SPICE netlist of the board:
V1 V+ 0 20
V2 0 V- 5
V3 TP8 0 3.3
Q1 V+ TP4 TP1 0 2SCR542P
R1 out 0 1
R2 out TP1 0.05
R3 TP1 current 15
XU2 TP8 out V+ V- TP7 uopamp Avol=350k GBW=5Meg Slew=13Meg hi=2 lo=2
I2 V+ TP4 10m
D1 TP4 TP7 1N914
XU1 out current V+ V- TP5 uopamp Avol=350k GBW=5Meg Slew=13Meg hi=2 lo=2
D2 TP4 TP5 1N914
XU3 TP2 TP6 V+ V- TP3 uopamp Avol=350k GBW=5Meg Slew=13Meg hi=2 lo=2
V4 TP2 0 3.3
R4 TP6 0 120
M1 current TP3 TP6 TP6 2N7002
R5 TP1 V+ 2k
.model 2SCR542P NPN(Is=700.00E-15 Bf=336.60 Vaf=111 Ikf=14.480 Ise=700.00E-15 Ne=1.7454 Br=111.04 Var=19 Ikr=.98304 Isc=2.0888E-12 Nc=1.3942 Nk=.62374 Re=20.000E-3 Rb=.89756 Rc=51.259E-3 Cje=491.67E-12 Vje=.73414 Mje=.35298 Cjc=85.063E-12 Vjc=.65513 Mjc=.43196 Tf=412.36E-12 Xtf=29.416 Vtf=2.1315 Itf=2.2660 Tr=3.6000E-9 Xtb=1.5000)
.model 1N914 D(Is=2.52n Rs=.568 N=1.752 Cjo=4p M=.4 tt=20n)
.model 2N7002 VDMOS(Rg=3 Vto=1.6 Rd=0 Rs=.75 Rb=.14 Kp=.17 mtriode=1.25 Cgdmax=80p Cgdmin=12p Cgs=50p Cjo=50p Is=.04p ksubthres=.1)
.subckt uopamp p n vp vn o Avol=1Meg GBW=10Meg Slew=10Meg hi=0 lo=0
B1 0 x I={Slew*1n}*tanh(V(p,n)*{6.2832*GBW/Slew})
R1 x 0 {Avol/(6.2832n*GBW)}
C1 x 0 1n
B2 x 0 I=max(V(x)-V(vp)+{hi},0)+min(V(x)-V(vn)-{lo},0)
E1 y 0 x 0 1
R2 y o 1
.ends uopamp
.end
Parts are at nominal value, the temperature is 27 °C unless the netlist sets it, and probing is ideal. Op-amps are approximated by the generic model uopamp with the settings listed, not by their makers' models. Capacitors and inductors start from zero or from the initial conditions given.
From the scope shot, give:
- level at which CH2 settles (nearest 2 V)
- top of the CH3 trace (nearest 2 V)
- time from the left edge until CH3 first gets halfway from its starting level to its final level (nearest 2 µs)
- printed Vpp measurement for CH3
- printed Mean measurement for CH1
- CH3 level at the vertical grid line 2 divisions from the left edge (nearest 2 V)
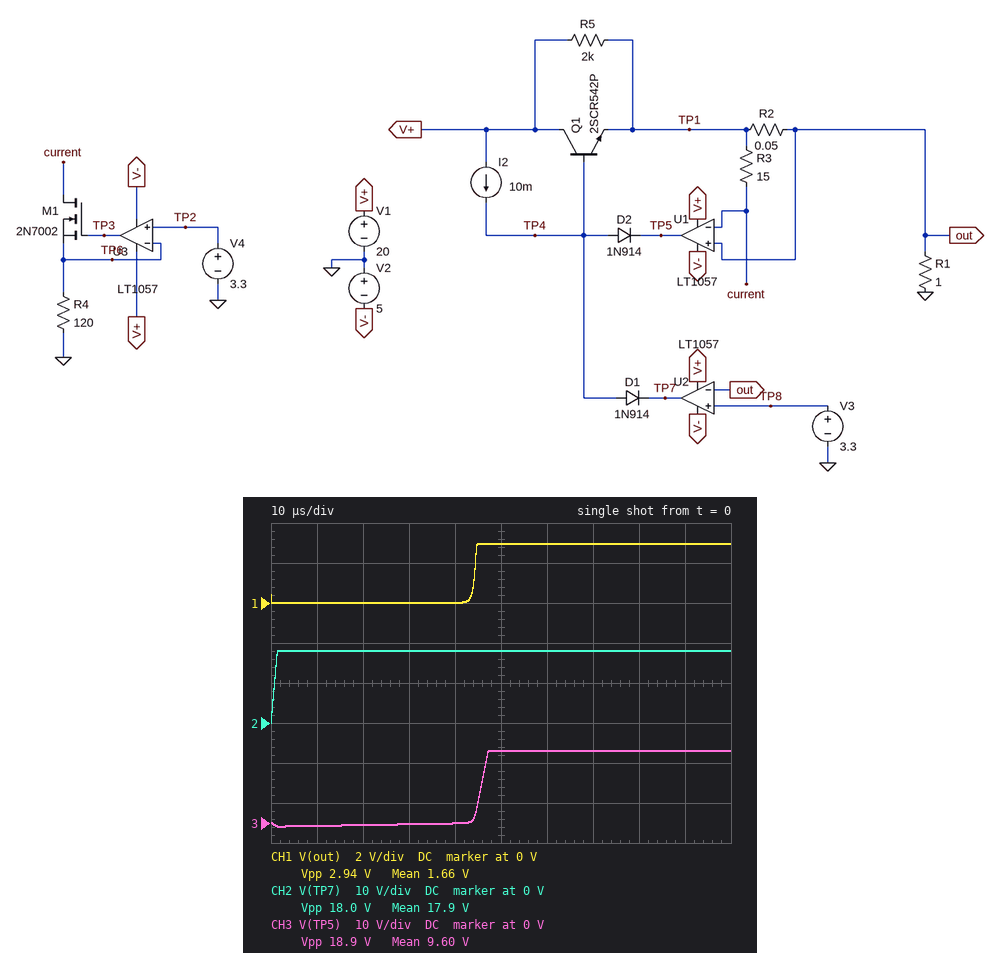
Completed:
18 V
18 V
46 µs
18.9 V
1.66 V
0 V
